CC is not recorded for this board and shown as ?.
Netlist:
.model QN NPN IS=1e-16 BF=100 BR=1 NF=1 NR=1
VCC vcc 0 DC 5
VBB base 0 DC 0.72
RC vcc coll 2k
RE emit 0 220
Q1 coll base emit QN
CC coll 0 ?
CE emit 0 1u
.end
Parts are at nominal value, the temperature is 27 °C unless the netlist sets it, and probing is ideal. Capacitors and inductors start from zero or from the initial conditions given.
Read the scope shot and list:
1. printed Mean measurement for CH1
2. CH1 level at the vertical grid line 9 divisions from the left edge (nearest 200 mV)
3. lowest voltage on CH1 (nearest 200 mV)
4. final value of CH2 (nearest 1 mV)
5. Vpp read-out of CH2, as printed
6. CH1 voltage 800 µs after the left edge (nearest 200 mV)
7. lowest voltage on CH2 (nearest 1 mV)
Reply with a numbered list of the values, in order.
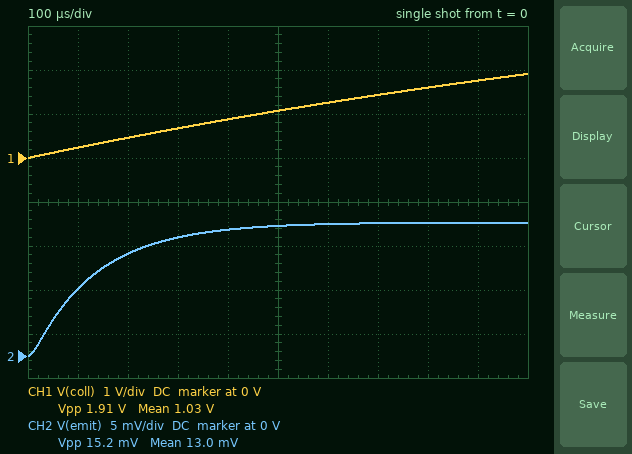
1. 1.03 V
2. 1.8 V
3. 0 V
4. 15 mV
5. 15.2 mV
6. 1.6 V
7. 0 V
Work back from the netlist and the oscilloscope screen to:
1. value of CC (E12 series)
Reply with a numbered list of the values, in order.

1. 1 µF
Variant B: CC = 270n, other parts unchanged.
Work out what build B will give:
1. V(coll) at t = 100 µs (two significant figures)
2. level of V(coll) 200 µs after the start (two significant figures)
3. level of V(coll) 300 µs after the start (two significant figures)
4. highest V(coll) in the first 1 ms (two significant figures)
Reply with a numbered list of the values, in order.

1. 810 mV
2. 1.5 V
3. 2.1 V
4. 4.1 V
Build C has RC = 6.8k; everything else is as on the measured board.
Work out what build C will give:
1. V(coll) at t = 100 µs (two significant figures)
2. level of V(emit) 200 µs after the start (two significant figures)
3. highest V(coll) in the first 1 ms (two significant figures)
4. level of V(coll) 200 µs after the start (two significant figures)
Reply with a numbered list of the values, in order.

1. 70 mV
2. 11 mV
3. 620 mV
4. 130 mV
